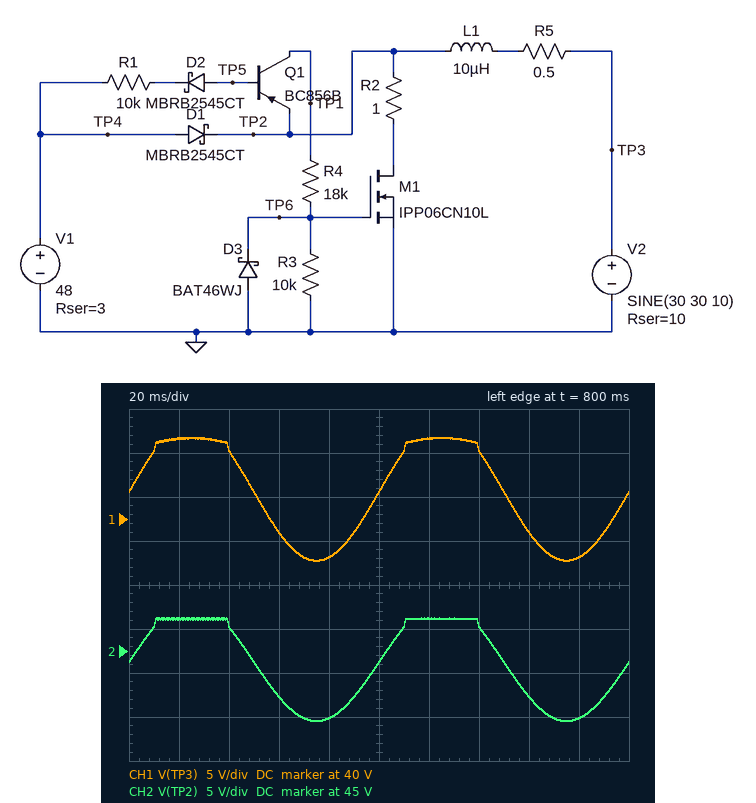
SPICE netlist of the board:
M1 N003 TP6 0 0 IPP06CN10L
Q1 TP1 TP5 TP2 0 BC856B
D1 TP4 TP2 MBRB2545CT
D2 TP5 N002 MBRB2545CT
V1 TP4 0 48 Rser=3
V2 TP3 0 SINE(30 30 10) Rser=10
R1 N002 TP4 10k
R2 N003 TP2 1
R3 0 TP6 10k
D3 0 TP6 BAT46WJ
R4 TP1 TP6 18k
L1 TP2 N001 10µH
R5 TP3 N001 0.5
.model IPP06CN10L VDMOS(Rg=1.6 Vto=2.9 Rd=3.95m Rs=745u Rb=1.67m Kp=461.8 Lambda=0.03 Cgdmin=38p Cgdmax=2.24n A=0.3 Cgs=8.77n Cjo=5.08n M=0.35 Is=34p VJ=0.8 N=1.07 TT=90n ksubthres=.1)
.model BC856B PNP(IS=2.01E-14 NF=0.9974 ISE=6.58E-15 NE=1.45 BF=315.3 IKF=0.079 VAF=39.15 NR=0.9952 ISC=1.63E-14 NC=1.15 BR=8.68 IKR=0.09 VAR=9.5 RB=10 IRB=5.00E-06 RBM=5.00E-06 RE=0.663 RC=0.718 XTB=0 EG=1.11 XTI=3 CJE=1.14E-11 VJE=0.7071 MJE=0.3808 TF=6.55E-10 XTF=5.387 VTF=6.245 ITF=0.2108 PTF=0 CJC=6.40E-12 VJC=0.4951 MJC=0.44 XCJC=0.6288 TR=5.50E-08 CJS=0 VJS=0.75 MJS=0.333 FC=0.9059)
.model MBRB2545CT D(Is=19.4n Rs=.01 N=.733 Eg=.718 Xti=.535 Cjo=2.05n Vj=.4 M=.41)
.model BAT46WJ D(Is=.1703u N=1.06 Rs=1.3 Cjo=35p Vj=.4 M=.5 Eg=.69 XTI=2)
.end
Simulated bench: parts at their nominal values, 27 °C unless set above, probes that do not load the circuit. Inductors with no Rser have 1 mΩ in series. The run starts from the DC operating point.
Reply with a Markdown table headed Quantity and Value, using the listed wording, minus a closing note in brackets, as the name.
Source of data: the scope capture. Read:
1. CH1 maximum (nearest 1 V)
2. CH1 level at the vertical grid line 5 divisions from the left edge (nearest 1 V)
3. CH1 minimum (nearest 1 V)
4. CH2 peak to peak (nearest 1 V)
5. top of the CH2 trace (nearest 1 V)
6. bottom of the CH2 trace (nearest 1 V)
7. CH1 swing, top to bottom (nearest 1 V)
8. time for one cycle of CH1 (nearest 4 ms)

| Quantity | Value |
|---|---|
| CH1 maximum | 49 V |
| CH1 level at the vertical grid line 5 divisions from the left edge | 43 V |
| CH1 minimum | 35 V |
| CH2 peak to peak | 12 V |
| top of the CH2 trace | 49 V |
| bottom of the CH2 trace | 37 V |
| CH1 swing, top to bottom | 14 V |
| time for one cycle of CH1 | 100 ms |
